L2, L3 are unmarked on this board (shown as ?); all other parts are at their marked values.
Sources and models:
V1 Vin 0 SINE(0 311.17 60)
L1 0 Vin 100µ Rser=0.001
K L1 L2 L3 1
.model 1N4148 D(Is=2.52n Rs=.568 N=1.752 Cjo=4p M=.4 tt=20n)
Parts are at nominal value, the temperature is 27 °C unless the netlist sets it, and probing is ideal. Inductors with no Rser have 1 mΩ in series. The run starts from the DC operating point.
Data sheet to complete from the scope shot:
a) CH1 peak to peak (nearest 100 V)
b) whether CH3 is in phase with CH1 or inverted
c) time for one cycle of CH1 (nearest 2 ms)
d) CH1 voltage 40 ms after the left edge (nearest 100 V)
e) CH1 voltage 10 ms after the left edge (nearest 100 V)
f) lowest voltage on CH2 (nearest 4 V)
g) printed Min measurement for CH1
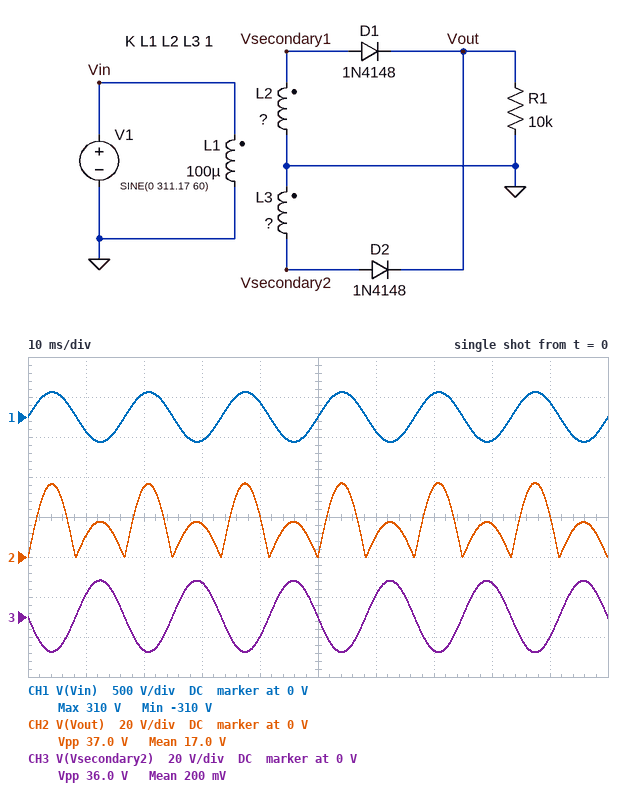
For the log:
600 V
inverted
16 ms
200 V
-200 V
0 V
-310 V
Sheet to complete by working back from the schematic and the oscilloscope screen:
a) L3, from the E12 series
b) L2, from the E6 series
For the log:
330 nH
1.5 µH
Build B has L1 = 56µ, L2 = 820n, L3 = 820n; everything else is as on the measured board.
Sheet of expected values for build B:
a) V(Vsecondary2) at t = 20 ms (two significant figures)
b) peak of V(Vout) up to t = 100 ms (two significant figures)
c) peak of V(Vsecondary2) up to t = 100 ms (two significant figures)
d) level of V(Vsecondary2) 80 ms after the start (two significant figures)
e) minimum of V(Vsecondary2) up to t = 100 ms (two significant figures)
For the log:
-35 V
38 V
39 V
36 V
-37 V
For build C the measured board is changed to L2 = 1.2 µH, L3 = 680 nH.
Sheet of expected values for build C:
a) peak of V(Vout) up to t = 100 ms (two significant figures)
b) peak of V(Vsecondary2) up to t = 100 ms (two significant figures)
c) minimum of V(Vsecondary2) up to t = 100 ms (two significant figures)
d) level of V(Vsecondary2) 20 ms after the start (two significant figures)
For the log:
33 V
26 V
-25 V
-24 V
